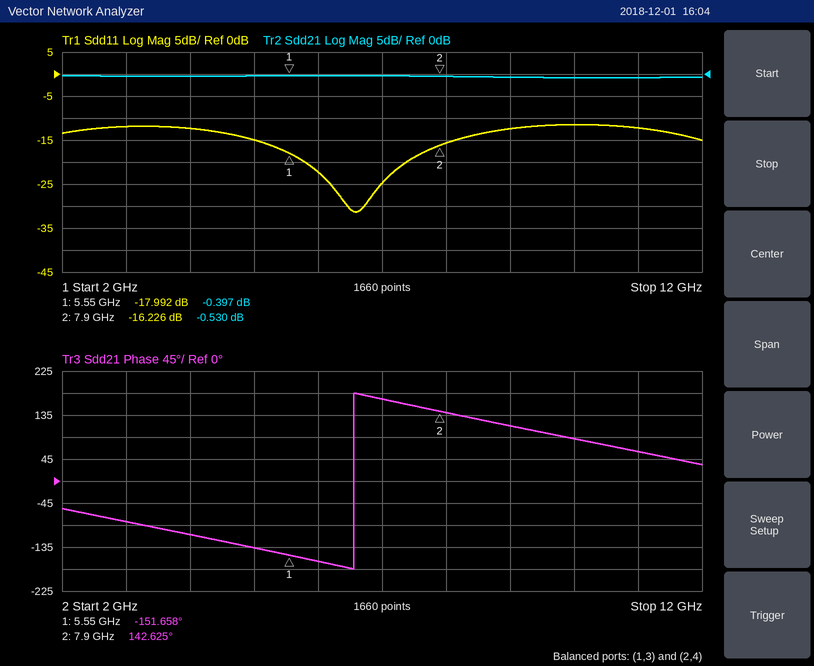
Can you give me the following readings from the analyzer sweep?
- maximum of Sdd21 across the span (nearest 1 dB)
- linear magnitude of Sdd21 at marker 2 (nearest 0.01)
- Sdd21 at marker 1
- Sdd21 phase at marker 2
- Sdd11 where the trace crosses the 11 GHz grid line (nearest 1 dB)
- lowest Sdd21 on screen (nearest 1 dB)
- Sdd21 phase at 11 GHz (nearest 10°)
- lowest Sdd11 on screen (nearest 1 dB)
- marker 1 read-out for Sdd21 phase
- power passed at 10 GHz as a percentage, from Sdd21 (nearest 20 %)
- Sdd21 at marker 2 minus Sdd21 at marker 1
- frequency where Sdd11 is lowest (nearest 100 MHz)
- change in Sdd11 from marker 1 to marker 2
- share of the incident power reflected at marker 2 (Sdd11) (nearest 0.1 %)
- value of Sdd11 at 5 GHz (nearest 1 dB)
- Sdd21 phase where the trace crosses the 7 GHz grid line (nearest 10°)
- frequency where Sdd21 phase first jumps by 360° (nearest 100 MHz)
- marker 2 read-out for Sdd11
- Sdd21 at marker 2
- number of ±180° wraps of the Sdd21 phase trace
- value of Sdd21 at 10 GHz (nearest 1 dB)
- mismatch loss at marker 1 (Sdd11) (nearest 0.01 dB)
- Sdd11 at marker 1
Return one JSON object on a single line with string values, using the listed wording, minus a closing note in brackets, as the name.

{"maximum of Sdd21 across the span": "0 dB", "linear magnitude of Sdd21 at marker 2": "0.94", "Sdd21 at marker 1": "-0.397 dB", "Sdd21 phase at marker 2": "142.625°", "Sdd11 where the trace crosses the 11 GHz grid line": "-12 dB", "lowest Sdd21 on screen": "-1 dB", "Sdd21 phase at 11 GHz": "60°", "lowest Sdd11 on screen": "-31 dB", "marker 1 read-out for Sdd21 phase": "-151.658°", "power passed at 10 GHz as a percentage, from Sdd21": "80 %", "Sdd21 at marker 2 minus Sdd21 at marker 1": "-0.133 dB", "frequency where Sdd11 is lowest": "6.6 GHz", "change in Sdd11 from marker 1 to marker 2": "1.766 dB", "share of the incident power reflected at marker 2 (Sdd11)": "2.4 %", "value of Sdd11 at 5 GHz": "-15 dB", "Sdd21 phase where the trace crosses the 7 GHz grid line": "170°", "frequency where Sdd21 phase first jumps by 360°": "6.6 GHz", "marker 2 read-out for Sdd11": "-16.226 dB", "Sdd21 at marker 2": "-0.530 dB", "number of ±180° wraps of the Sdd21 phase trace": "1", "value of Sdd21 at 10 GHz": "-1 dB", "mismatch loss at marker 1 (Sdd11)": "0.07 dB", "Sdd11 at marker 1": "-17.992 dB"}
